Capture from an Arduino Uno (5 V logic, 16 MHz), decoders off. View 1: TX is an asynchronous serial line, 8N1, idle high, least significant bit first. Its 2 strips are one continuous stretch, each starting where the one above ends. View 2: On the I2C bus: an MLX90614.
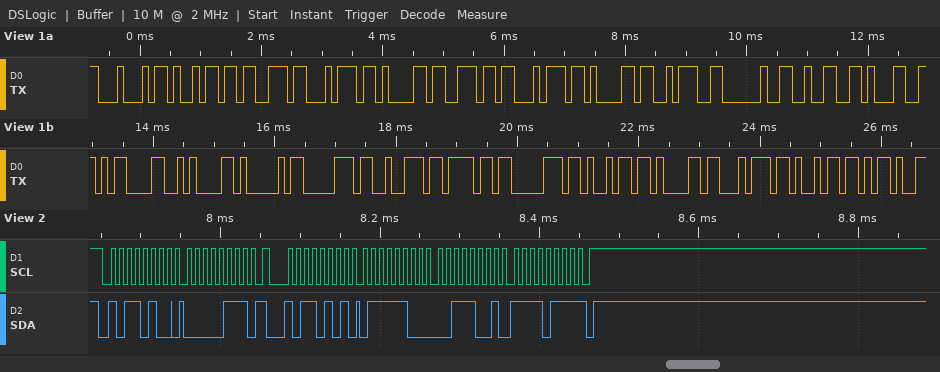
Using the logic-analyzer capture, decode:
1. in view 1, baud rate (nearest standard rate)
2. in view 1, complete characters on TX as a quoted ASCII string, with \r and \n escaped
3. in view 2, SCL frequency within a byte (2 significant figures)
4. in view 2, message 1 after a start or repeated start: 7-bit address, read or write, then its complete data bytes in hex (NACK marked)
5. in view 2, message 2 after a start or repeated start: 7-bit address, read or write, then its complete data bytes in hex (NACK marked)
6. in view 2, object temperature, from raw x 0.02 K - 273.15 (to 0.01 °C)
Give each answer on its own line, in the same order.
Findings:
9600 baud
"Distanta: 21\r\nApropiati-"
100 kHz
0x5A write: 07
0x5A read: 7C 39 F7 NACK
21.17 °C
